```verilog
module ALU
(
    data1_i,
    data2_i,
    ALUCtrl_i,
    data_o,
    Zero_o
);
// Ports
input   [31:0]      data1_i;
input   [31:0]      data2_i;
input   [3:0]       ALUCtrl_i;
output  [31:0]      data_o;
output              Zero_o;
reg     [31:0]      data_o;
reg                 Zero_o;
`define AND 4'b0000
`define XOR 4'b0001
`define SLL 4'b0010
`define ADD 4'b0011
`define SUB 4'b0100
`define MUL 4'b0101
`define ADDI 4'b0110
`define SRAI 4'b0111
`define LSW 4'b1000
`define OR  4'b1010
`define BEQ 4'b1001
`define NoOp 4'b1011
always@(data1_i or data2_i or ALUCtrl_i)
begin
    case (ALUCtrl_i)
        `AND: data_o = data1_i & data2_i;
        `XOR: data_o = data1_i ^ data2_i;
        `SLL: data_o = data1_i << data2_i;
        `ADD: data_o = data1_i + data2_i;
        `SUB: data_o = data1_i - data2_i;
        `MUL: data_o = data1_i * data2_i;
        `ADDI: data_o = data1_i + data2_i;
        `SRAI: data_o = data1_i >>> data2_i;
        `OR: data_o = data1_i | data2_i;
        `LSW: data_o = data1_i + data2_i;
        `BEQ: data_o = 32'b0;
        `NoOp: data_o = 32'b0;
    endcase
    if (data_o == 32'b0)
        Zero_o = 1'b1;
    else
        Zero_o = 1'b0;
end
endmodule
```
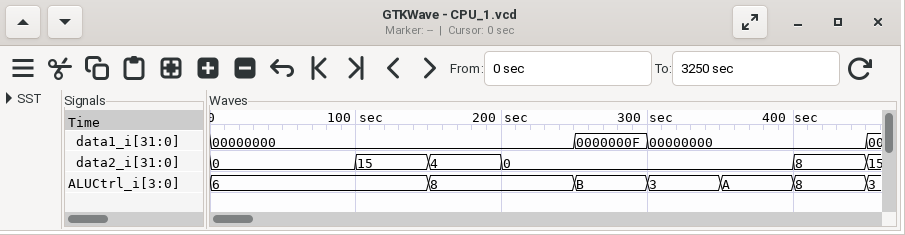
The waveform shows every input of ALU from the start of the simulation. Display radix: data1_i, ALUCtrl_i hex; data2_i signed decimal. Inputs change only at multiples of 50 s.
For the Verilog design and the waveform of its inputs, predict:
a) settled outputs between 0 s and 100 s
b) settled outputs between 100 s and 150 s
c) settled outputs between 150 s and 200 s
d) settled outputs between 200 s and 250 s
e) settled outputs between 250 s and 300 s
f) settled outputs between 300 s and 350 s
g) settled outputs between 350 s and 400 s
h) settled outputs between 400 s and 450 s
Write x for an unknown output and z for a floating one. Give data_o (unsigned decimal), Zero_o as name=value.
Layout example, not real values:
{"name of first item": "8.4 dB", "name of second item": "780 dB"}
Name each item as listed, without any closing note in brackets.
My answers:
{"settled outputs between 0 s and 100 s": "data_o=0, Zero_o=1", "settled outputs between 100 s and 150 s": "data_o=15, Zero_o=0", "settled outputs between 150 s and 200 s": "data_o=4, Zero_o=0", "settled outputs between 200 s and 250 s": "data_o=0, Zero_o=1", "settled outputs between 250 s and 300 s": "data_o=0, Zero_o=1", "settled outputs between 300 s and 350 s": "data_o=0, Zero_o=1", "settled outputs between 350 s and 400 s": "data_o=0, Zero_o=1", "settled outputs between 400 s and 450 s": "data_o=8, Zero_o=0"}
